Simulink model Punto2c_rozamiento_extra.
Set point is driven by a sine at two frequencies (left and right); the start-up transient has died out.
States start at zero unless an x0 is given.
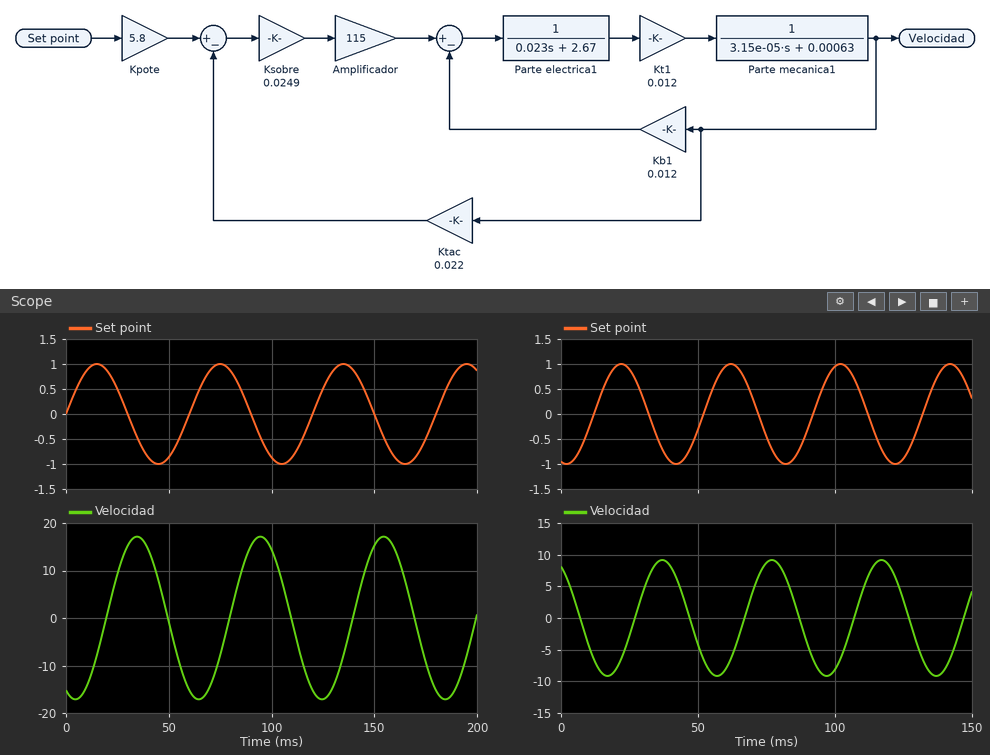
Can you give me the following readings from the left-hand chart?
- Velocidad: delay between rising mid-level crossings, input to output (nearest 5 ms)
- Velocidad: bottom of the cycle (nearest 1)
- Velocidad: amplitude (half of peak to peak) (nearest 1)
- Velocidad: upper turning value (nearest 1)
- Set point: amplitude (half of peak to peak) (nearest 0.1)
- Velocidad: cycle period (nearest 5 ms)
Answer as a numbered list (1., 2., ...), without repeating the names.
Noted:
1. 20 ms
2. -17
3. 17
4. 17
5. 1.0
6. 60 ms
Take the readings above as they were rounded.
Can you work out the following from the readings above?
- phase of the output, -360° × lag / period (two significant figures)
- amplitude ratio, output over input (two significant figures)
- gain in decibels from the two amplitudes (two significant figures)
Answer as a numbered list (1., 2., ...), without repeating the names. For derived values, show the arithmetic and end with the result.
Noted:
1. -360 × 20 / 60 = -120°
2. 17 / 1 = 17
3. 20 log10(17 / 1) = 25 dB
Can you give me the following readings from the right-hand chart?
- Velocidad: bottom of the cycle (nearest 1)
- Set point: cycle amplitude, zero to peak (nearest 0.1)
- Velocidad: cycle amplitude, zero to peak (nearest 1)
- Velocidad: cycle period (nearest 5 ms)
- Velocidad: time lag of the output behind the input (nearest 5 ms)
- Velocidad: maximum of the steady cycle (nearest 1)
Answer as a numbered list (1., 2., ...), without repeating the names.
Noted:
1. -9
2. 1.0
3. 9
4. 40 ms
5. 15 ms
6. 9
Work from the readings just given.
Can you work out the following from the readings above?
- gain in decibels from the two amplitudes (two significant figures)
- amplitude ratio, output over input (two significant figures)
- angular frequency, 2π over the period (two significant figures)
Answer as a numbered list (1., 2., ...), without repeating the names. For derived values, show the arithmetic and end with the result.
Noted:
1. 20 log10(9 / 1) = 19 dB
2. 9 / 1 = 9.0
3. 2π / 40 = 0.16 rad/ms
